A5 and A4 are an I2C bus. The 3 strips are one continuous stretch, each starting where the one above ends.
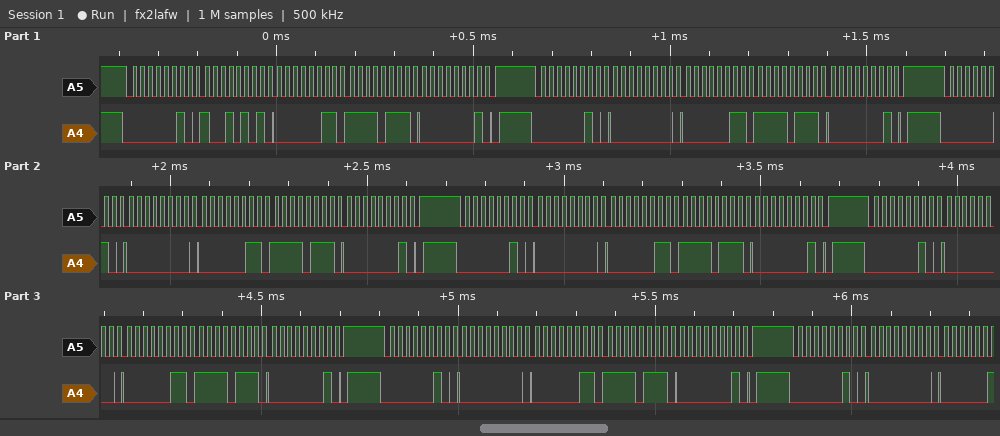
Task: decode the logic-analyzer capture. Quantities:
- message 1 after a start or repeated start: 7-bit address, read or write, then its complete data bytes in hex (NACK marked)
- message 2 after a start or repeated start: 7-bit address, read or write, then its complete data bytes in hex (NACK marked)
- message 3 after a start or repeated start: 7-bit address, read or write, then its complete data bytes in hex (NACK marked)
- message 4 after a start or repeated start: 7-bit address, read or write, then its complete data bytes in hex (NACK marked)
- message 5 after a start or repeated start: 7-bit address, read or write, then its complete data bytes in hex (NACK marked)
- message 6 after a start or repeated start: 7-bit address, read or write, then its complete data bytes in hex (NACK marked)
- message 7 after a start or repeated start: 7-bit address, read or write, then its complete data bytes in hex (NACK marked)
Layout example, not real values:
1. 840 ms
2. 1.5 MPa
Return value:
1. 0x01 write: 95 03 F7 01
2. 0x01 write: 00 03 F7 01
3. 0x01 write: 00 03 F7 01
4. 0x01 write: 00 03 F7 01
5. 0x01 write: 00 03 F7 01
6. 0x01 write: 00 03 F7 01
7. 0x01 write: 00
